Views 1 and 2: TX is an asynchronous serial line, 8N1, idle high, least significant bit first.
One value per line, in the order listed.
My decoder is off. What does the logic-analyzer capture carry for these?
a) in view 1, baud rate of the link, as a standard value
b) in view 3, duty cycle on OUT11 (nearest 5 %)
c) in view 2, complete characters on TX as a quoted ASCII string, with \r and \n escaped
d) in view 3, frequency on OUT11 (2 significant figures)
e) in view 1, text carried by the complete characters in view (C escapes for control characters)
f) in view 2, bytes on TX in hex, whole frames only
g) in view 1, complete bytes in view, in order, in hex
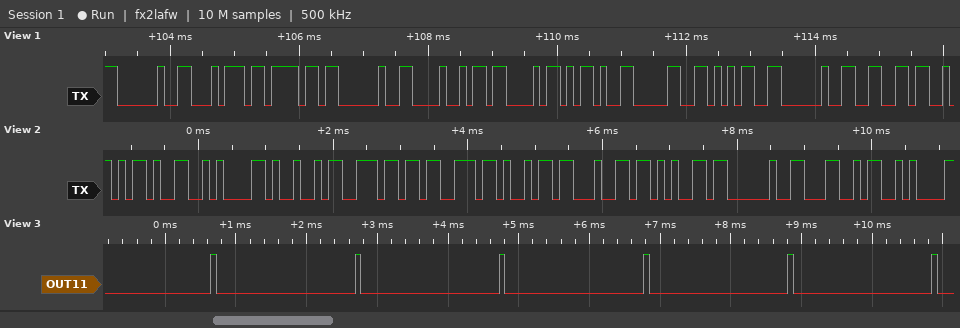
9600 baud
5 %
"-\nInside L\n"
490 Hz
" to HC-05 f"
0x2D 0x0A 0x49 0x6E 0x73 0x69 0x64 0x65 0x20 0x4C 0x0A
20 74 6F 20 48 43 2D 30 35 20 66
